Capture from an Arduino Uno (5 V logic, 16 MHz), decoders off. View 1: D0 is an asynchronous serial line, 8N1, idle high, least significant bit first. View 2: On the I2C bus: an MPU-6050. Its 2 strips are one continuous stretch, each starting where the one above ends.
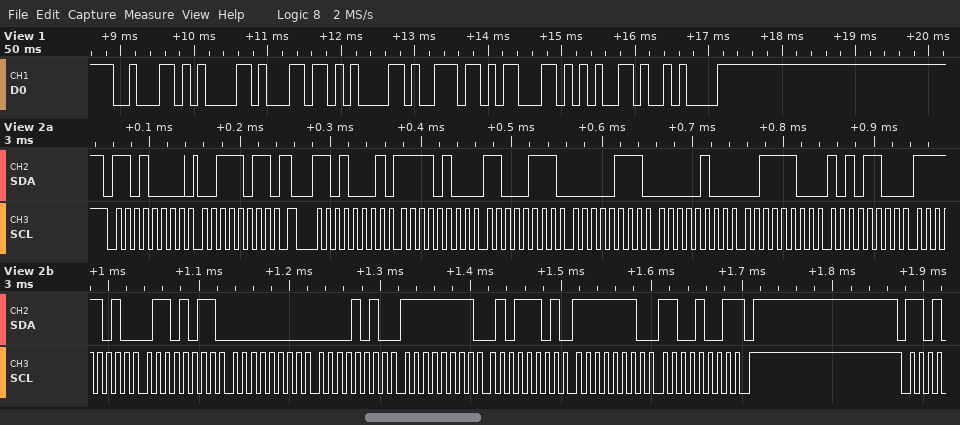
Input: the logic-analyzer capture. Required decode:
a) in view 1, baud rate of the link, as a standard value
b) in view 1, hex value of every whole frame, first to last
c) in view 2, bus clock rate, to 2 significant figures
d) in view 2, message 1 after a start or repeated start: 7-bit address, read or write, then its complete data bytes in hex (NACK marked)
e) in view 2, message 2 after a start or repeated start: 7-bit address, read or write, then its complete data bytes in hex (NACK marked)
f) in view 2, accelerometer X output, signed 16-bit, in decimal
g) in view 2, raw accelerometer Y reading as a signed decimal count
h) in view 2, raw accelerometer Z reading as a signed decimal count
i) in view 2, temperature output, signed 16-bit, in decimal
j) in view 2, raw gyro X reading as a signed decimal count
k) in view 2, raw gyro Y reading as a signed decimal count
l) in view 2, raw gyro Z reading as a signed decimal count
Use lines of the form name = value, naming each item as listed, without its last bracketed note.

in view 1, baud rate of the link, as a standard value = 9600 baud
in view 1, hex value of every whole frame, first to last = 62 61 6C 61 6E 63 65 0A
in view 2, bus clock rate, to 2 significant figures = 100 kHz
in view 2, message 1 after a start or repeated start: 7-bit address, read or write, then its complete data bytes in hex = 0x68 write: 3B
in view 2, message 2 after a start or repeated start: 7-bit address, read or write, then its complete data bytes in hex = 0x68 read: F4 C7 07 04 3C AC FA 6B 00 0A FF 5D FE C9 NACK
in view 2, accelerometer X output, signed 16-bit, in decimal = -2873
in view 2, raw accelerometer Y reading as a signed decimal count = 1796
in view 2, raw accelerometer Z reading as a signed decimal count = 15532
in view 2, temperature output, signed 16-bit, in decimal = -1429
in view 2, raw gyro X reading as a signed decimal count = 10
in view 2, raw gyro Y reading as a signed decimal count = -163
in view 2, raw gyro Z reading as a signed decimal count = -311
